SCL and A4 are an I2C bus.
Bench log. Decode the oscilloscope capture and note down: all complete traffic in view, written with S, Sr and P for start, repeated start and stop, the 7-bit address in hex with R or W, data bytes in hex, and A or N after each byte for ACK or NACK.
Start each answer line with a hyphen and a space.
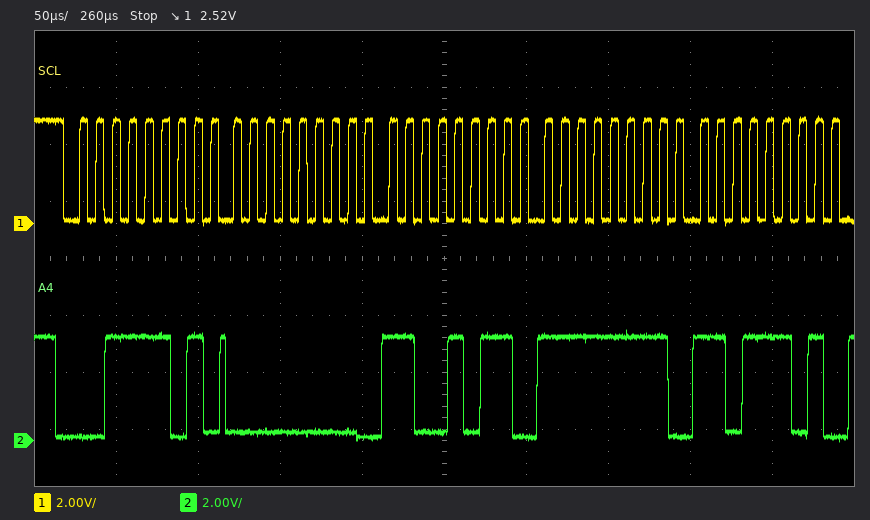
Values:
- S 1ER A 00 A CB A FF A DD A
